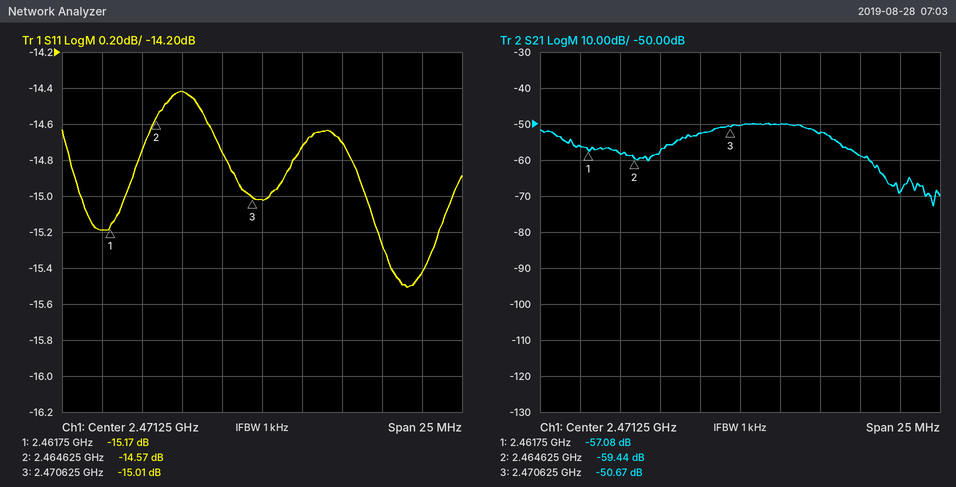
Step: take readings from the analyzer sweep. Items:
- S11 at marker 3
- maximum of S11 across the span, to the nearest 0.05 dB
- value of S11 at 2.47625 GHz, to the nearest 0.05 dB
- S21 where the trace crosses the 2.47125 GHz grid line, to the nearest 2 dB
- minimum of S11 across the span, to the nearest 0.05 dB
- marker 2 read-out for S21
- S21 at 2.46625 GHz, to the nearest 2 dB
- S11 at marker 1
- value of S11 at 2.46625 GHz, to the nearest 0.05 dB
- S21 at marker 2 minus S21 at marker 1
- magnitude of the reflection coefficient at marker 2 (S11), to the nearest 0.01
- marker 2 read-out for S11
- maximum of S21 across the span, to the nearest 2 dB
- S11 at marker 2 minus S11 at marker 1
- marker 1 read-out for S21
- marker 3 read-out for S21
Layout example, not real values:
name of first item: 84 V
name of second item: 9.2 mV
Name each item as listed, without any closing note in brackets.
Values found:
S11 at marker 3: -15.01 dB
maximum of S11 across the span, to the nearest 0.05 dB: -14.40 dB
value of S11 at 2.47625 GHz, to the nearest 0.05 dB: -14.70 dB
S21 where the trace crosses the 2.47125 GHz grid line, to the nearest 2 dB: -50 dB
minimum of S11 across the span, to the nearest 0.05 dB: -15.50 dB
marker 2 read-out for S21: -59.44 dB
S21 at 2.46625 GHz, to the nearest 2 dB: -58 dB
S11 at marker 1: -15.17 dB
value of S11 at 2.46625 GHz, to the nearest 0.05 dB: -14.40 dB
S21 at marker 2 minus S21 at marker 1: -2.36 dB
magnitude of the reflection coefficient at marker 2 (S11), to the nearest 0.01: 0.19
marker 2 read-out for S11: -14.57 dB
maximum of S21 across the span, to the nearest 2 dB: -50 dB
S11 at marker 2 minus S11 at marker 1: 0.60 dB
marker 1 read-out for S21: -57.08 dB
marker 3 read-out for S21: -50.67 dB
